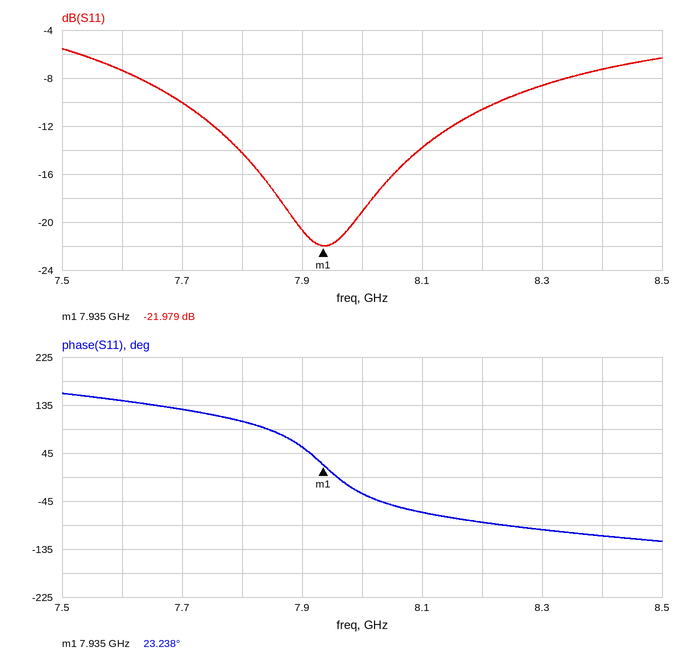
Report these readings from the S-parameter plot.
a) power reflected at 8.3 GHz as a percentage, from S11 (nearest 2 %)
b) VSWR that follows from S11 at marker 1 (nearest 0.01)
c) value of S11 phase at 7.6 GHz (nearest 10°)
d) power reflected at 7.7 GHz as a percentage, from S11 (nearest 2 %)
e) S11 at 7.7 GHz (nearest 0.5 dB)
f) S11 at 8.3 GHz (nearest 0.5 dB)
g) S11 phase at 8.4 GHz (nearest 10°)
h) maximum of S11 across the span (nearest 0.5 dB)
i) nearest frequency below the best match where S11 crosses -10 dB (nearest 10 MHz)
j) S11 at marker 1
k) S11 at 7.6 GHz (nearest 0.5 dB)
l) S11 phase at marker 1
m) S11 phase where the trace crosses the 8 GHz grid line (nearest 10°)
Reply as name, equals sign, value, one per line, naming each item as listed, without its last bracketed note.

power reflected at 8.3 GHz as a percentage, from S11 = 14 %
VSWR that follows from S11 at marker 1 = 1.17
value of S11 phase at 7.6 GHz = 140°
power reflected at 7.7 GHz as a percentage, from S11 = 10 %
S11 at 7.7 GHz = -10.0 dB
S11 at 8.3 GHz = -8.5 dB
S11 phase at 8.4 GHz = -110°
maximum of S11 across the span = -5.5 dB
nearest frequency below the best match where S11 crosses -10 dB = 7.70 GHz
S11 at marker 1 = -21.979 dB
S11 at 7.6 GHz = -7.5 dB
S11 phase at marker 1 = 23.238°
S11 phase where the trace crosses the 8 GHz grid line = -30°
